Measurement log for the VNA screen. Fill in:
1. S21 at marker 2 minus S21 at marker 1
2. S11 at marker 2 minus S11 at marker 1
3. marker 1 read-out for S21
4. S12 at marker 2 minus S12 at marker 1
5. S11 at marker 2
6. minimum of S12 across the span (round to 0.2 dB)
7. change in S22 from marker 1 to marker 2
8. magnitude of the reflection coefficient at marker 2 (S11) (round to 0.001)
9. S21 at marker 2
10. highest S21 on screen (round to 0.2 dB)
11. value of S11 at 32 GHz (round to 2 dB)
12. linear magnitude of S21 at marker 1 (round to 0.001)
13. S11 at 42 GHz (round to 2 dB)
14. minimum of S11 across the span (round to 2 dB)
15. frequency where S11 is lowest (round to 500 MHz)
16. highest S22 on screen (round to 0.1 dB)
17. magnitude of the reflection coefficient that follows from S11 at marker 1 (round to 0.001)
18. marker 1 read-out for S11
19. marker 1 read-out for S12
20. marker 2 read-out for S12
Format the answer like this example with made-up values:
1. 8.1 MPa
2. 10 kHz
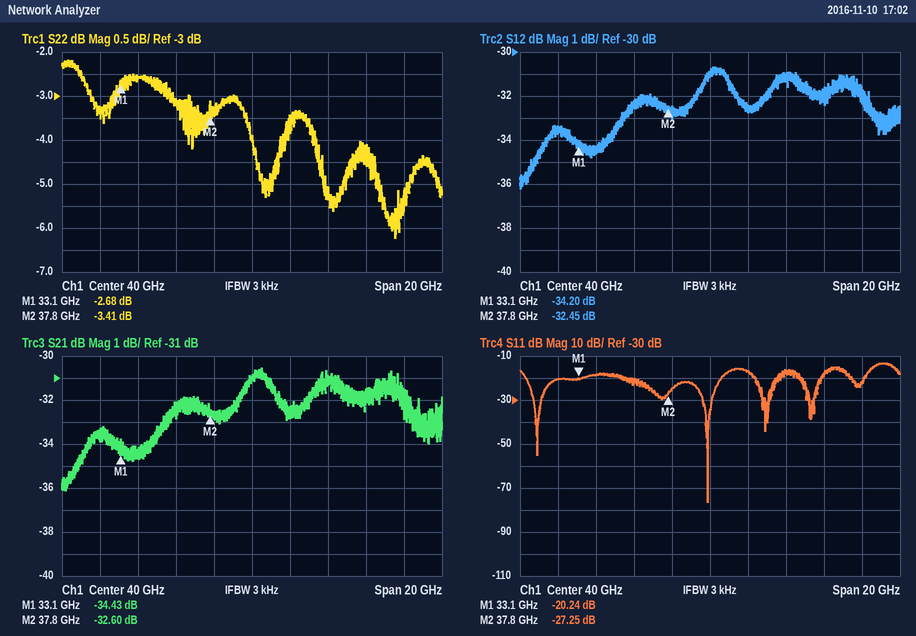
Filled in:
1. 1.83 dB
2. -7.01 dB
3. -34.43 dB
4. 1.75 dB
5. -27.25 dB
6. -36.2 dB
7. -0.73 dB
8. 0.043
9. -32.60 dB
10. -30.6 dB
11. -20 dB
12. 0.019
13. -16 dB
14. -76 dB
15. 40.0 GHz
16. -2.2 dB
17. 0.097
18. -20.24 dB
19. -34.20 dB
20. -32.45 dB
